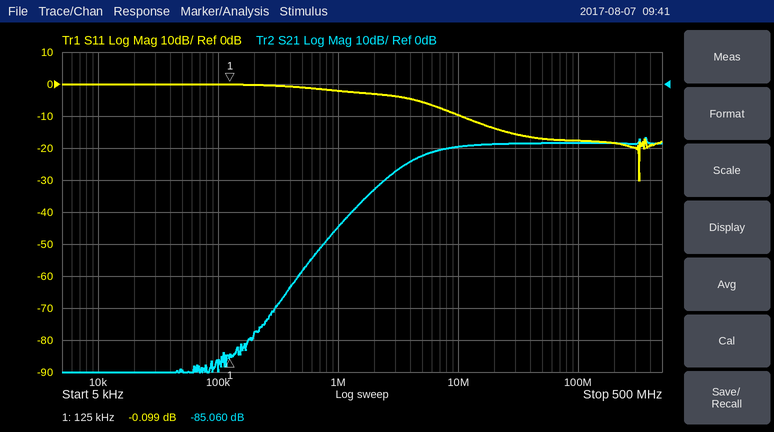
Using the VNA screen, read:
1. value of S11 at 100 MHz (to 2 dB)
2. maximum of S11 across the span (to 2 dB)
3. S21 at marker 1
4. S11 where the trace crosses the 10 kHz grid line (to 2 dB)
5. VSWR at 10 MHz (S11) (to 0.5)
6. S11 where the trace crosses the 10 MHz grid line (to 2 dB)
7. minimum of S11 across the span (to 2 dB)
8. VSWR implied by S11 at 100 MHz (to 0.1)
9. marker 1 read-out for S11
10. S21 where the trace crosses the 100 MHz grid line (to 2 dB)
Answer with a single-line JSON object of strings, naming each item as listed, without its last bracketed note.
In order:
{"value of S11 at 100 MHz": "-18 dB", "maximum of S11 across the span": "0 dB", "S21 at marker 1": "-85.060 dB", "S11 where the trace crosses the 10 kHz grid line": "0 dB", "VSWR at 10 MHz (S11)": "2.0", "S11 where the trace crosses the 10 MHz grid line": "-10 dB", "minimum of S11 across the span": "-30 dB", "VSWR implied by S11 at 100 MHz": "1.3", "marker 1 read-out for S11": "-0.099 dB", "S21 where the trace crosses the 100 MHz grid line": "-18 dB"}
